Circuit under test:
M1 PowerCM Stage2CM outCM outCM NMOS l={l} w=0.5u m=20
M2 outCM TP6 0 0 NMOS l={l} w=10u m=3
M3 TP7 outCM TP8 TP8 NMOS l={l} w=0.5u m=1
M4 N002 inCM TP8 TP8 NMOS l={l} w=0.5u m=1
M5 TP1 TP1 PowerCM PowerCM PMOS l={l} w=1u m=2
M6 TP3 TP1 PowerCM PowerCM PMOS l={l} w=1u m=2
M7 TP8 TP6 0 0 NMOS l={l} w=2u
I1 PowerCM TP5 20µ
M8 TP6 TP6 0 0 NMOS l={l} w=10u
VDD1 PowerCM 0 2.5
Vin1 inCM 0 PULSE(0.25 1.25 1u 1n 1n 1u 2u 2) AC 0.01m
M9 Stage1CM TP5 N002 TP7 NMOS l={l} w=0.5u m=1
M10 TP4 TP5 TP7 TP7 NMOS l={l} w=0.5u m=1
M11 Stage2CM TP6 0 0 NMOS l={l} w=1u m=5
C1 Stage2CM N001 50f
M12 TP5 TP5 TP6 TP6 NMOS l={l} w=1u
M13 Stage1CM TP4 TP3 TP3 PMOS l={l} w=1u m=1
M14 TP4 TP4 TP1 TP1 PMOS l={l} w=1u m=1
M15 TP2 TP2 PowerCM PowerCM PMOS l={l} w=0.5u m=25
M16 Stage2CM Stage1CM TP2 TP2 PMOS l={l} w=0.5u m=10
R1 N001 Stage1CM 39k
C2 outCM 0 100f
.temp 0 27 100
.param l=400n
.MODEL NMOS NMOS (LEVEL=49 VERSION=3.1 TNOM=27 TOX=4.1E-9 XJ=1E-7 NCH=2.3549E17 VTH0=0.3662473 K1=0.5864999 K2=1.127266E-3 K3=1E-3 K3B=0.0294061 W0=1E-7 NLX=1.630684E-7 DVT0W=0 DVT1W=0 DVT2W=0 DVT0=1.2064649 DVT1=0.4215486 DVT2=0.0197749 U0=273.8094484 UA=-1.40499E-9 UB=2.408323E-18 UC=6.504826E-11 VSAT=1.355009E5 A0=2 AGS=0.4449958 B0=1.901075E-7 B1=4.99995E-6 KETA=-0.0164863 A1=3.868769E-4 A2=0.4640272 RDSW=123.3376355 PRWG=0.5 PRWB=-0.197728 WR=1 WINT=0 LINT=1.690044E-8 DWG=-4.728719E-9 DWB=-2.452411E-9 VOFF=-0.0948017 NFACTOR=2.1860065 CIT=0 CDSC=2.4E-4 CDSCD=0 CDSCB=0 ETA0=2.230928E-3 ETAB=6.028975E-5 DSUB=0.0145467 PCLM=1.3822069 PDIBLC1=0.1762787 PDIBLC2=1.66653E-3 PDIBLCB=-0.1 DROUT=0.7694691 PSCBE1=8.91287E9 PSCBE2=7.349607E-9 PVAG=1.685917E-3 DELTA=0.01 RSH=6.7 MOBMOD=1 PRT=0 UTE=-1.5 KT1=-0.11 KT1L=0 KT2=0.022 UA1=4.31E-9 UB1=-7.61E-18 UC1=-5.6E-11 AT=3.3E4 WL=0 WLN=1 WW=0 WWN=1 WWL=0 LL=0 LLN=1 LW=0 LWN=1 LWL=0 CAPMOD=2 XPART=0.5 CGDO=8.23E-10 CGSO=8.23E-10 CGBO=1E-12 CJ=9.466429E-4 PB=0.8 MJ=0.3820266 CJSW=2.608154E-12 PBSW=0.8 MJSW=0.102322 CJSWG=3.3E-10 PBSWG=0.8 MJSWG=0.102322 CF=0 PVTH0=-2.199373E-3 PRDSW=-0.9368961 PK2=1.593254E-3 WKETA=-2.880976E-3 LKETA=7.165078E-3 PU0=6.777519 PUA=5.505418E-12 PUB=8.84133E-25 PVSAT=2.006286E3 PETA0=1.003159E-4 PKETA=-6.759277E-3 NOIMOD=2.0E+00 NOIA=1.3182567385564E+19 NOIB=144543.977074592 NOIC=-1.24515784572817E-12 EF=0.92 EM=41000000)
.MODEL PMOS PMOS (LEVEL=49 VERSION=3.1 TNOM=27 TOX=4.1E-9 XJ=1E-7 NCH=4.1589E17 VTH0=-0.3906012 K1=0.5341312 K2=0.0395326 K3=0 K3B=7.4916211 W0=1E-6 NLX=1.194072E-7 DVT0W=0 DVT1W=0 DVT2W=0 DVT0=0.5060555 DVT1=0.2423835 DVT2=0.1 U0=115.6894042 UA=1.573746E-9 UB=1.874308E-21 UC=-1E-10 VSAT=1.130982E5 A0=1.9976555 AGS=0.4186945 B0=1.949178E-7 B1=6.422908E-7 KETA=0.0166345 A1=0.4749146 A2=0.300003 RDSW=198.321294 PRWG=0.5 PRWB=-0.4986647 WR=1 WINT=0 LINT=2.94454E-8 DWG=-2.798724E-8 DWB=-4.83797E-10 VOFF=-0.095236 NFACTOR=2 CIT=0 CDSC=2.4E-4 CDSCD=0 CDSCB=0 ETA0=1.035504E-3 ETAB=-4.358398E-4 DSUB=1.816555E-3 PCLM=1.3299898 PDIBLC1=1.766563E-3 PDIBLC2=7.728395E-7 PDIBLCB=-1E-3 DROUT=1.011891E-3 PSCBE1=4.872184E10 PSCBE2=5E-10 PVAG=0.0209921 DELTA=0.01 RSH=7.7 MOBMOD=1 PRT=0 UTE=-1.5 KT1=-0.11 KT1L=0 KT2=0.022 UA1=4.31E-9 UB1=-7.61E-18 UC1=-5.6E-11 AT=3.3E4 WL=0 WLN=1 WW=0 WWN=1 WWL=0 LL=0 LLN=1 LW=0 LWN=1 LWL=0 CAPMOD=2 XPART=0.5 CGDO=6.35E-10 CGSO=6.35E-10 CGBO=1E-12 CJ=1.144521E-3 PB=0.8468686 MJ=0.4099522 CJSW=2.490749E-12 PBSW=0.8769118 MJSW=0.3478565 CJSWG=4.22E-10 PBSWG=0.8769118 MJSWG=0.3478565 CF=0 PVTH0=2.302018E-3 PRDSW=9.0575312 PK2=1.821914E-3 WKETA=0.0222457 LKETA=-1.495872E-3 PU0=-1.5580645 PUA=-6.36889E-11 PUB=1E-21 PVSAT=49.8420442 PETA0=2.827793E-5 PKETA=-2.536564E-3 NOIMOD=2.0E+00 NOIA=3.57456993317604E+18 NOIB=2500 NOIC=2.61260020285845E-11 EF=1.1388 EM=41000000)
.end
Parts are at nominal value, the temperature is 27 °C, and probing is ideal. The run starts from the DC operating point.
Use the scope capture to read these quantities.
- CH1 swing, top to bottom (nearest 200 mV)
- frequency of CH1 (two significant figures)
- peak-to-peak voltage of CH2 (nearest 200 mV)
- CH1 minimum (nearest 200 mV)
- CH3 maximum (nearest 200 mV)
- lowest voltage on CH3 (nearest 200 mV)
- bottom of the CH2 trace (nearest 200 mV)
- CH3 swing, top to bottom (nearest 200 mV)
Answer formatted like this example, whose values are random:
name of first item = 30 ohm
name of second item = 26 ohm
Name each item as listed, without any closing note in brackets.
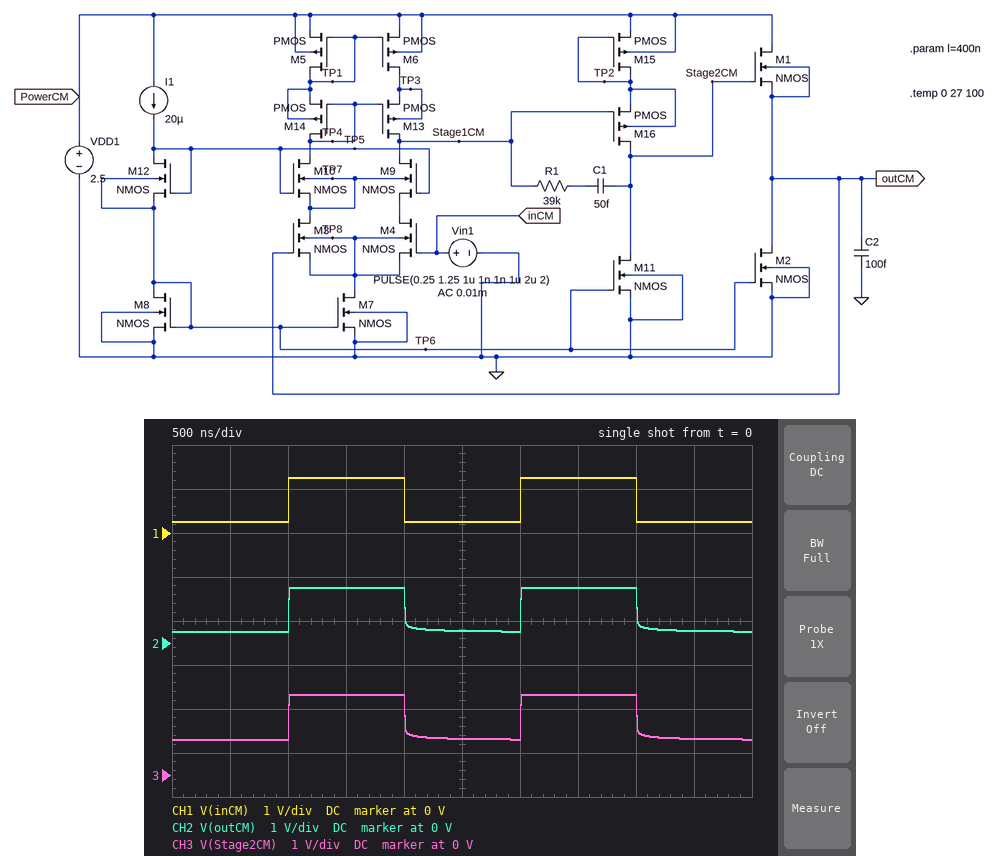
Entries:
CH1 swing, top to bottom = 1.0 V
frequency of CH1 = 500 kHz
peak-to-peak voltage of CH2 = 1.0 V
CH1 minimum = 200 mV
CH3 maximum = 1.8 V
lowest voltage on CH3 = 800 mV
bottom of the CH2 trace = 200 mV
CH3 swing, top to bottom = 1.0 V
